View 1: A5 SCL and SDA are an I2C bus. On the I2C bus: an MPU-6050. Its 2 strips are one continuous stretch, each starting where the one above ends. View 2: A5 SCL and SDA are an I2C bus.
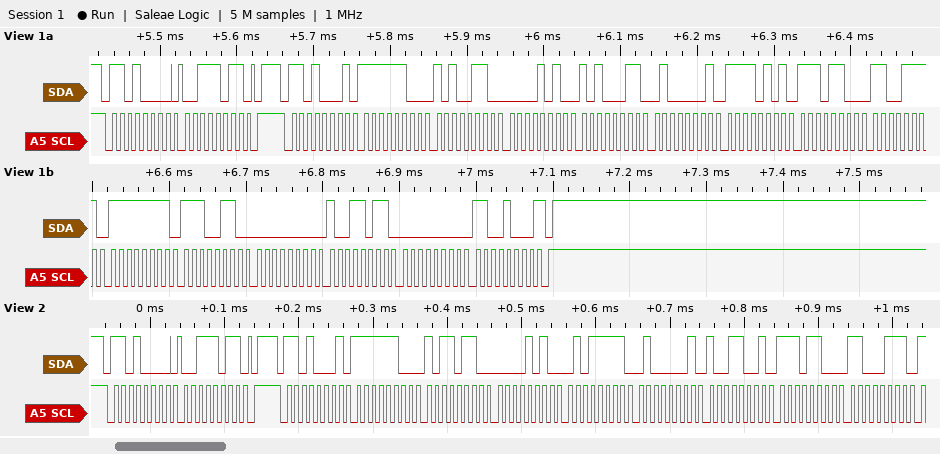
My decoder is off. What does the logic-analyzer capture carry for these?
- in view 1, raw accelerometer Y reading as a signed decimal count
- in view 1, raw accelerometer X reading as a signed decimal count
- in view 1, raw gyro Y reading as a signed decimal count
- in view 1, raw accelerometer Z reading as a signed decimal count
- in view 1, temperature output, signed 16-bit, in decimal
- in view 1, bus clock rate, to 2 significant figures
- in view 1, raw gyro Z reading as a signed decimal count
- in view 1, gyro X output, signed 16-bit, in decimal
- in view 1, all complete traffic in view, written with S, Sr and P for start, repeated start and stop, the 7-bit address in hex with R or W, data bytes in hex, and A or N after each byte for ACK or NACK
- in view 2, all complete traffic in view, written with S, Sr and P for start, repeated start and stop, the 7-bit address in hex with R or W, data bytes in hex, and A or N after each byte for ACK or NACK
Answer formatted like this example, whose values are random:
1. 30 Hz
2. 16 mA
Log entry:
1. 2723
2. -858
3. 155
4. 16885
5. -4913
6. 100 kHz
7. 200
8. -26
9. S 68W A 3B A P S 68R A FC A A6 A 0A A A3 A 41 A F5 A EC A CF A FF A E6 A 00 A 9B A 00 A C8 N P
10. S 68W A 3B A P S 68R A FC A B6 A 0A A 5F A 41 A 99 A EC A C7 A
